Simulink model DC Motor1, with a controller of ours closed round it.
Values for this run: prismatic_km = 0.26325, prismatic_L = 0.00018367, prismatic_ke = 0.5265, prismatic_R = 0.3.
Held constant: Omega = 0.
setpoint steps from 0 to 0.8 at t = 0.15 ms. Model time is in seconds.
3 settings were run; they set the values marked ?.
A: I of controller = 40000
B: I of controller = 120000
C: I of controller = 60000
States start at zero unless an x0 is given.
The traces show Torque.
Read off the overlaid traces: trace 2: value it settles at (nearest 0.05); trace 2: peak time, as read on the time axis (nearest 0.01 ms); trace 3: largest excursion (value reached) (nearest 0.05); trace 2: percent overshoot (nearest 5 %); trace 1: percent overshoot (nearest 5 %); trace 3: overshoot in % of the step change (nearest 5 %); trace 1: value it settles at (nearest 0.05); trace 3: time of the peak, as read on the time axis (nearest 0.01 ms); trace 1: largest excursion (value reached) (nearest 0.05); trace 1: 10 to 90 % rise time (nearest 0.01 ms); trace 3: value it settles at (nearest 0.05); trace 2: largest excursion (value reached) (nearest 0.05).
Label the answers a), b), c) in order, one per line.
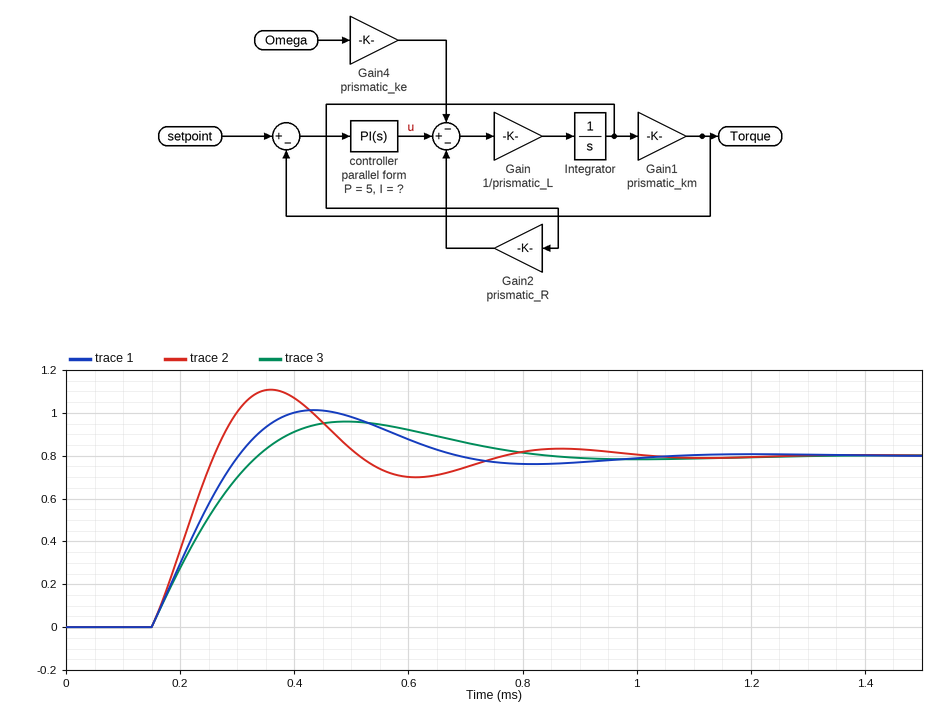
a) 0.80
b) 0.36 ms
c) 0.95
d) 40 %
e) 25 %
f) 20 %
g) 0.80
h) 0.49 ms
i) 1.00
j) 0.12 ms
k) 0.80
l) 1.10
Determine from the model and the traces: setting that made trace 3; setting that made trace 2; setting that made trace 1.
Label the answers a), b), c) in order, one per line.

a) A
b) B
c) C
